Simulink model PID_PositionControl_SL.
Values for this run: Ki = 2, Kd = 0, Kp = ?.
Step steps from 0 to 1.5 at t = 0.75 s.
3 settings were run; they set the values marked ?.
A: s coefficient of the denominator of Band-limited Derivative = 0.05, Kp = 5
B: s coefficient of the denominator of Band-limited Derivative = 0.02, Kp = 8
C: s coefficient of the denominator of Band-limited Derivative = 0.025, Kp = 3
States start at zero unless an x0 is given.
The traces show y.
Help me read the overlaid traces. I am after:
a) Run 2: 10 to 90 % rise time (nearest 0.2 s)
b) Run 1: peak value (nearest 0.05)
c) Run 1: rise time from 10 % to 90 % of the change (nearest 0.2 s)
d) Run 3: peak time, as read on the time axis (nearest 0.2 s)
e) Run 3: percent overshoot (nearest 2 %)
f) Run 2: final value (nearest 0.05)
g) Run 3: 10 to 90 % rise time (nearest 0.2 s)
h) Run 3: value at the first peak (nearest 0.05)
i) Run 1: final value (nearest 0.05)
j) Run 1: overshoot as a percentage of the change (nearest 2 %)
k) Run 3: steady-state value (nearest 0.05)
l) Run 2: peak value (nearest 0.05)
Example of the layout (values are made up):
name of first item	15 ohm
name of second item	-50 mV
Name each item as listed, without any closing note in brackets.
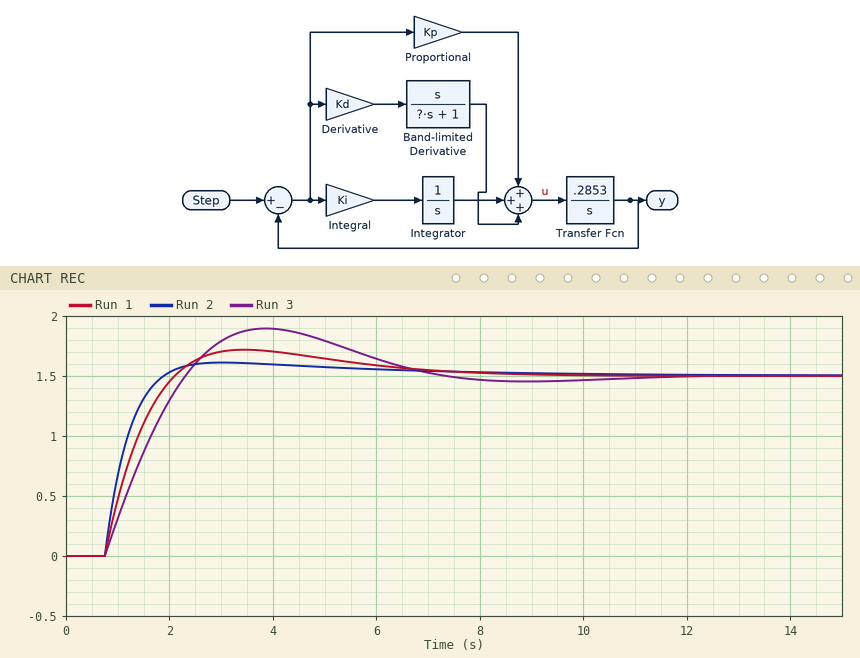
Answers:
Run 2: 10 to 90 % rise time	0.8 s
Run 1: peak value	1.70
Run 1: rise time from 10 % to 90 % of the change	1.0 s
Run 3: peak time, as read on the time axis	3.8 s
Run 3: percent overshoot	26 %
Run 2: final value	1.50
Run 3: 10 to 90 % rise time	1.2 s
Run 3: value at the first peak	1.90
Run 1: final value	1.50
Run 1: overshoot as a percentage of the change	14 %
Run 3: steady-state value	1.50
Run 2: peak value	1.60
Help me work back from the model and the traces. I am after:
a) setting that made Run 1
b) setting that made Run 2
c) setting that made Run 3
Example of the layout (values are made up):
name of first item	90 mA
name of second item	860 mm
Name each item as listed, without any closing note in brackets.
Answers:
setting that made Run 1	A
setting that made Run 2	B
setting that made Run 3	C
